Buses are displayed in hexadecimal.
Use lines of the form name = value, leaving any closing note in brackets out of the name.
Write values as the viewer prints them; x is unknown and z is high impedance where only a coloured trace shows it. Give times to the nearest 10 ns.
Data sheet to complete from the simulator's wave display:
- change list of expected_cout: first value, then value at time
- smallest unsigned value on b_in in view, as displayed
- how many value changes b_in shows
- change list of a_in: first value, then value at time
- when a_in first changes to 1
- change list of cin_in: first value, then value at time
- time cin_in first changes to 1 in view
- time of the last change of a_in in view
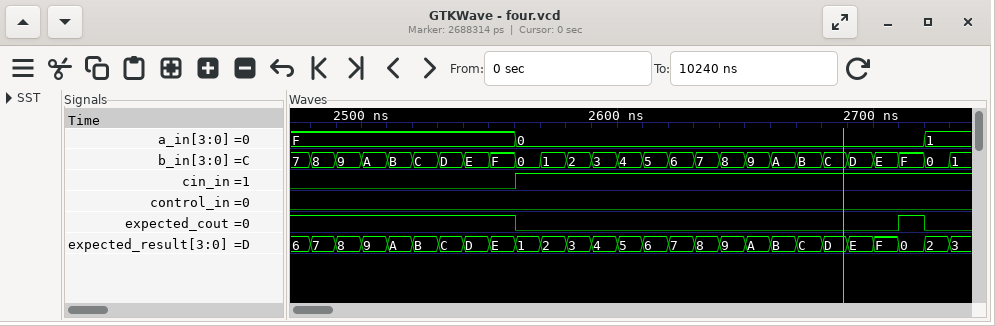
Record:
change list of expected_cout: first value, then value at time = 1, 0 at 2560 ns, 1 at 2710 ns, 0 at 2720 ns
smallest unsigned value on b_in in view, as displayed = 0
how many value changes b_in shows = 26
change list of a_in: first value, then value at time = F, 0 at 2560 ns, 1 at 2720 ns
when a_in first changes to 1 = 2720 ns
change list of cin_in: first value, then value at time = 0, 1 at 2560 ns
time cin_in first changes to 1 in view = 2560 ns
time of the last change of a_in in view = 2720 ns
